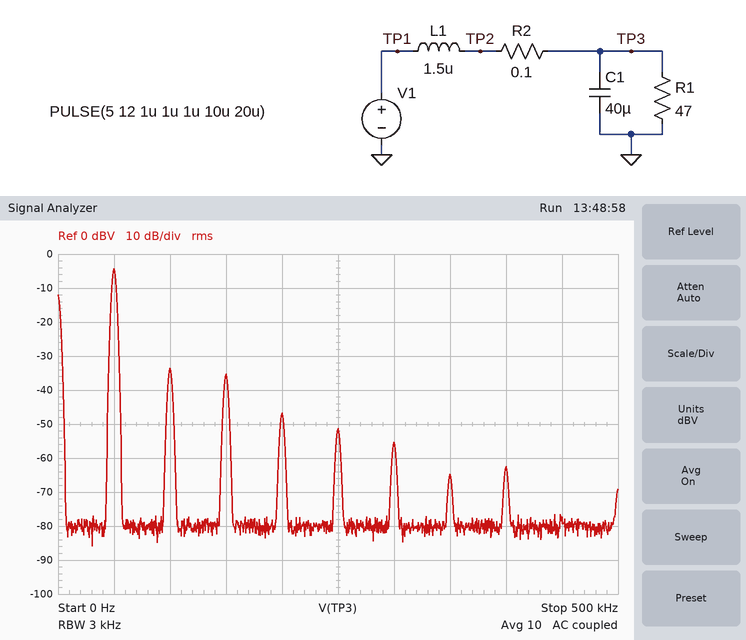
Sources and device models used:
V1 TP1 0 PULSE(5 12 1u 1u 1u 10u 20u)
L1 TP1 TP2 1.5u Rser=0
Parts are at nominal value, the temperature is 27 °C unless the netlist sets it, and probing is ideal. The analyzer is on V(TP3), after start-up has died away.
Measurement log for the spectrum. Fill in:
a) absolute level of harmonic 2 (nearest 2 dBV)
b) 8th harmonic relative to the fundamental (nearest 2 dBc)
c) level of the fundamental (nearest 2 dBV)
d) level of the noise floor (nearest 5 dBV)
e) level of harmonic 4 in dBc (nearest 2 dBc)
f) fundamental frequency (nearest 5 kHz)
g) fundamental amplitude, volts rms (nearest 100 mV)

-34 dBV
-58 dBc
-4 dBV
-80 dBV
-42 dBc
50 kHz
600 mV
